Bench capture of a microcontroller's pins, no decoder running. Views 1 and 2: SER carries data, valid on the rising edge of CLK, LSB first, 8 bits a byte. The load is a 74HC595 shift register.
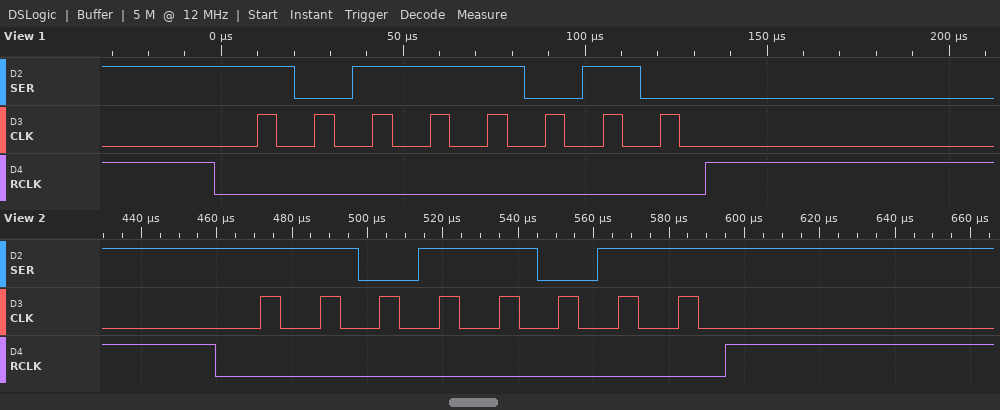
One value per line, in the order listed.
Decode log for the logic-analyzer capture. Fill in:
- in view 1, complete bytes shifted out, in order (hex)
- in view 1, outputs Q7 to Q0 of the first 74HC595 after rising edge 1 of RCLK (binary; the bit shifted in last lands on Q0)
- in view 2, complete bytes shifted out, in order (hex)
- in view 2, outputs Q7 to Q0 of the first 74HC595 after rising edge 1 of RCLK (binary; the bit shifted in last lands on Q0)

5D
10111010
DB
11011011
